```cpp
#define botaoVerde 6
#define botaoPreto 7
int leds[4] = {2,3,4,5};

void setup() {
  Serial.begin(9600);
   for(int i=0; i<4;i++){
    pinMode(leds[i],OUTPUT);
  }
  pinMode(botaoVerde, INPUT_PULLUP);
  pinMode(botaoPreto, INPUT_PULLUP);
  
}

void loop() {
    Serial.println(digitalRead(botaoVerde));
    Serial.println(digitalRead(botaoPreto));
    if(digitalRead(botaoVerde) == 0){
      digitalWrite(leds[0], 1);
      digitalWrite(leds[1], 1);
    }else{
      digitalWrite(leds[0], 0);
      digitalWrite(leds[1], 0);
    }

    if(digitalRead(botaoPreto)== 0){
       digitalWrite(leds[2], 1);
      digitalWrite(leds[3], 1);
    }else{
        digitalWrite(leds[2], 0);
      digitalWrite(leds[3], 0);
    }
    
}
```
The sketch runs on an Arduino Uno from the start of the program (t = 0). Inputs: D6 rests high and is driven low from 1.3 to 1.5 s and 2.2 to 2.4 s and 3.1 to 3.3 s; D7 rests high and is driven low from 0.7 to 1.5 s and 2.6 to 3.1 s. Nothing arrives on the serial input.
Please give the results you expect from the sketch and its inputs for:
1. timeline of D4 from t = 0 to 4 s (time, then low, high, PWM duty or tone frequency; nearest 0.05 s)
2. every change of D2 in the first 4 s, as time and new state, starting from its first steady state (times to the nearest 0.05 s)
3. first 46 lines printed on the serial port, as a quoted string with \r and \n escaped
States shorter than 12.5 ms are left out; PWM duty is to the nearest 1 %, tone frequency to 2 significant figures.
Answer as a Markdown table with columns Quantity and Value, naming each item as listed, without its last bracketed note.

| Quantity | Value |
|---|---|
| timeline of D4 from t = 0 to 4 s | 0 s low; 0.7 s high; 1.5 s low; 2.6 s high; 3.1 s low |
| every change of D2 in the first 4 s, as time and new state, starting from its first steady state | 0 s low; 1.3 s high; 1.5 s low; 2.2 s high; 2.4 s low; 3.1 s high; 3.3 s low |
| first 46 lines printed on the serial port, as a quoted string with \r and \n escaped | "1\r\n1\r\n1\r\n1\r\n1\r\n1\r\n1\r\n1\r\n1\r\n1\r\n1\r\n1\r\n1\r\n1\r\n1\r\n1\r\n1\r\n1\r\n1\r\n1\r\n1\r\n1\r\n1\r\n1\r\n1\r\n1\r\n1\r\n1\r\n1\r\n1\r\n1\r\n1\r\n1\r\n1\r\n1\r\n1\r\n1\r\n1\r\n1\r\n1\r\n1\r\n1\r\n1\r\n1\r\n1\r\n1\r\n" |
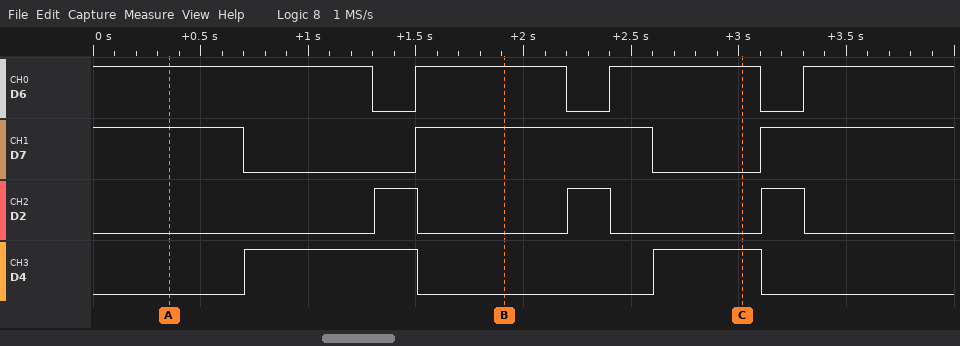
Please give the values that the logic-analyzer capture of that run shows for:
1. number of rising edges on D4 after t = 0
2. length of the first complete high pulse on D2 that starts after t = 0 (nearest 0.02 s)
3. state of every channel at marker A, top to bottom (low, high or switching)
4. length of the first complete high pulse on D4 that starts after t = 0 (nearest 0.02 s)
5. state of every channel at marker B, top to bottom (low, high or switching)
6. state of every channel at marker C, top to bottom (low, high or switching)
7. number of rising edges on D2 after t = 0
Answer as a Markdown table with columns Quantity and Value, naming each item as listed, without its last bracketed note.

| Quantity | Value |
|---|---|
| number of rising edges on D4 after t = 0 | 2 |
| length of the first complete high pulse on D2 that starts after t = 0 | 0.20 s |
| state of every channel at marker A, top to bottom | D6 high, D7 high, D2 low, D4 low |
| length of the first complete high pulse on D4 that starts after t = 0 | 0.80 s |
| state of every channel at marker B, top to bottom | D6 high, D7 high, D2 low, D4 low |
| state of every channel at marker C, top to bottom | D6 high, D7 low, D2 low, D4 high |
| number of rising edges on D2 after t = 0 | 3 |
